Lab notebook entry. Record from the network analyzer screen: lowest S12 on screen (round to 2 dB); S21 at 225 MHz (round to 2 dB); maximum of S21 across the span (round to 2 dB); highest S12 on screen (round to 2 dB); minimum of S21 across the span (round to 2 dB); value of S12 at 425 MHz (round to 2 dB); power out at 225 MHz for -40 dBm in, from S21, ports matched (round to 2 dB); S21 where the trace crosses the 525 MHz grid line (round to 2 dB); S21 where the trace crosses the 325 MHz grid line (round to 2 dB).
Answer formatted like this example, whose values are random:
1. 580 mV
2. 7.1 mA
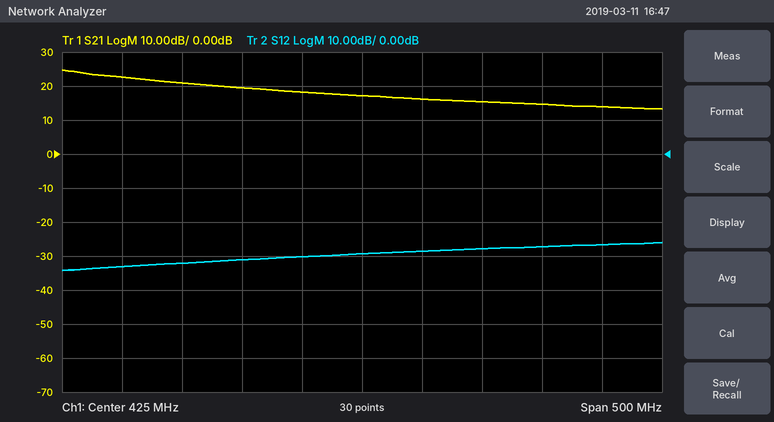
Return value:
1. -34 dB
2. 22 dB
3. 24 dB
4. -26 dB
5. 14 dB
6. -30 dB
7. -18 dBm
8. 16 dB
9. 20 dB
